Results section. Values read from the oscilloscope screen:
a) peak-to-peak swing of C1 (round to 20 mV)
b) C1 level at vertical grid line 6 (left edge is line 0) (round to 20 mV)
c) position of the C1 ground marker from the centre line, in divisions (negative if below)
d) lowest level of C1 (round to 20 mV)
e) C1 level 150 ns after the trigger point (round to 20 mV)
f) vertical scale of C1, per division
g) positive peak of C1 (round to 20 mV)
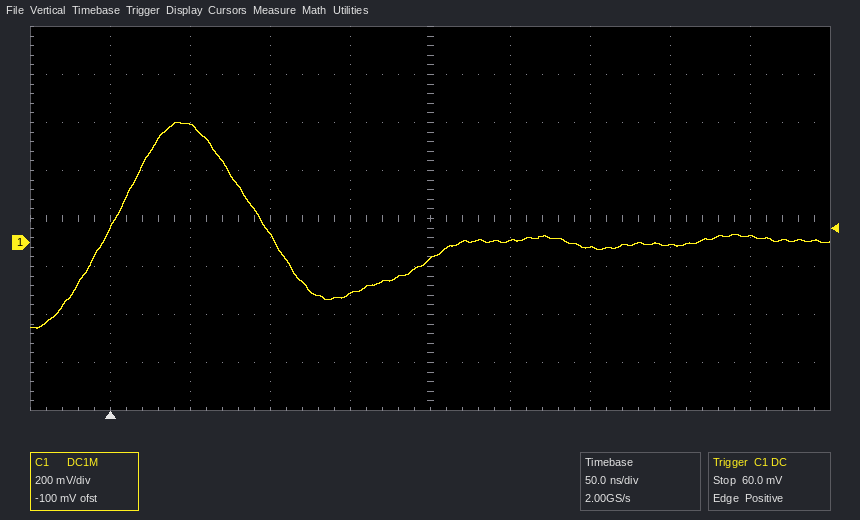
860 mV
0 mV
-0.5 div
-360 mV
-220 mV
200 mV
500 mV
